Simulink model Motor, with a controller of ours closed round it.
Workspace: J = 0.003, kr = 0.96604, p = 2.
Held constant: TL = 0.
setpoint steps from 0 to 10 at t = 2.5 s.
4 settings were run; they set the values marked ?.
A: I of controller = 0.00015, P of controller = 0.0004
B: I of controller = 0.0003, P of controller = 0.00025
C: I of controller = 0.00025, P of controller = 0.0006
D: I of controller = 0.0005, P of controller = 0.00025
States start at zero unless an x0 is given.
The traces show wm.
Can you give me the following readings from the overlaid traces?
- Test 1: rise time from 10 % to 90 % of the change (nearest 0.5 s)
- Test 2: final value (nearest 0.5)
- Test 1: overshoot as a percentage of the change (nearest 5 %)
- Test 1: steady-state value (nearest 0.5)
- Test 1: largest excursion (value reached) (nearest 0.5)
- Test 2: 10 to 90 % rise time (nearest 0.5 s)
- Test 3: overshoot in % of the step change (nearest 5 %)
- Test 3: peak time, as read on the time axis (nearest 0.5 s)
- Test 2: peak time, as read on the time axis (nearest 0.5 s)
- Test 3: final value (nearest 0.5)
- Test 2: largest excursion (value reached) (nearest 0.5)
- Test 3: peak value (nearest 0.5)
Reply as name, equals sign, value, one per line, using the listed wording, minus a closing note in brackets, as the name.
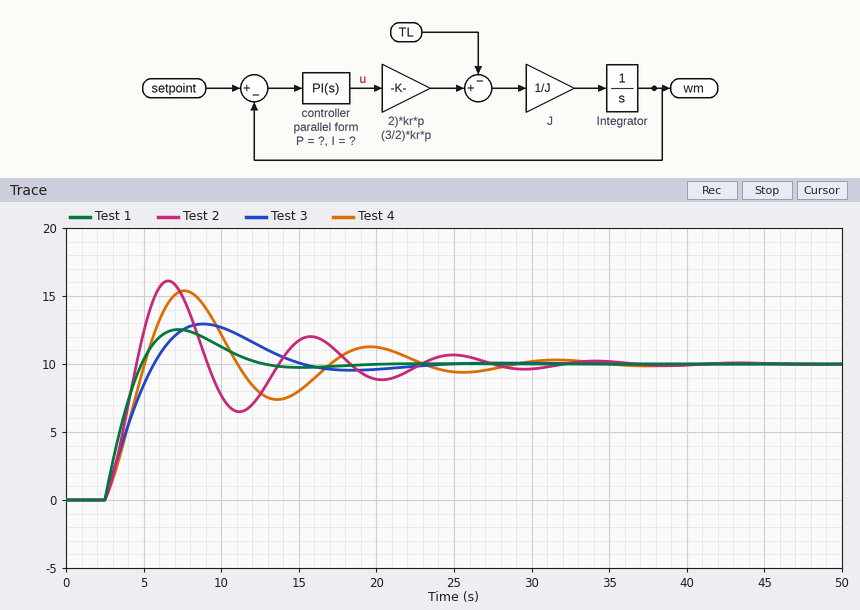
Test 1: rise time from 10 % to 90 % of the change = 2.0 s
Test 2: final value = 10.0
Test 1: overshoot as a percentage of the change = 25 %
Test 1: steady-state value = 10.0
Test 1: largest excursion (value reached) = 12.5
Test 2: 10 to 90 % rise time = 1.5 s
Test 3: overshoot in % of the step change = 30 %
Test 3: peak time, as read on the time axis = 9.0 s
Test 2: peak time, as read on the time axis = 6.5 s
Test 3: final value = 10.0
Test 2: largest excursion (value reached) = 16.0
Test 3: peak value = 13.0
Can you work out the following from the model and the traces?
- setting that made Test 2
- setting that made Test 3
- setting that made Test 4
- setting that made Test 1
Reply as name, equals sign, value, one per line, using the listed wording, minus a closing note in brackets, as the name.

setting that made Test 2 = D
setting that made Test 3 = A
setting that made Test 4 = B
setting that made Test 1 = C
